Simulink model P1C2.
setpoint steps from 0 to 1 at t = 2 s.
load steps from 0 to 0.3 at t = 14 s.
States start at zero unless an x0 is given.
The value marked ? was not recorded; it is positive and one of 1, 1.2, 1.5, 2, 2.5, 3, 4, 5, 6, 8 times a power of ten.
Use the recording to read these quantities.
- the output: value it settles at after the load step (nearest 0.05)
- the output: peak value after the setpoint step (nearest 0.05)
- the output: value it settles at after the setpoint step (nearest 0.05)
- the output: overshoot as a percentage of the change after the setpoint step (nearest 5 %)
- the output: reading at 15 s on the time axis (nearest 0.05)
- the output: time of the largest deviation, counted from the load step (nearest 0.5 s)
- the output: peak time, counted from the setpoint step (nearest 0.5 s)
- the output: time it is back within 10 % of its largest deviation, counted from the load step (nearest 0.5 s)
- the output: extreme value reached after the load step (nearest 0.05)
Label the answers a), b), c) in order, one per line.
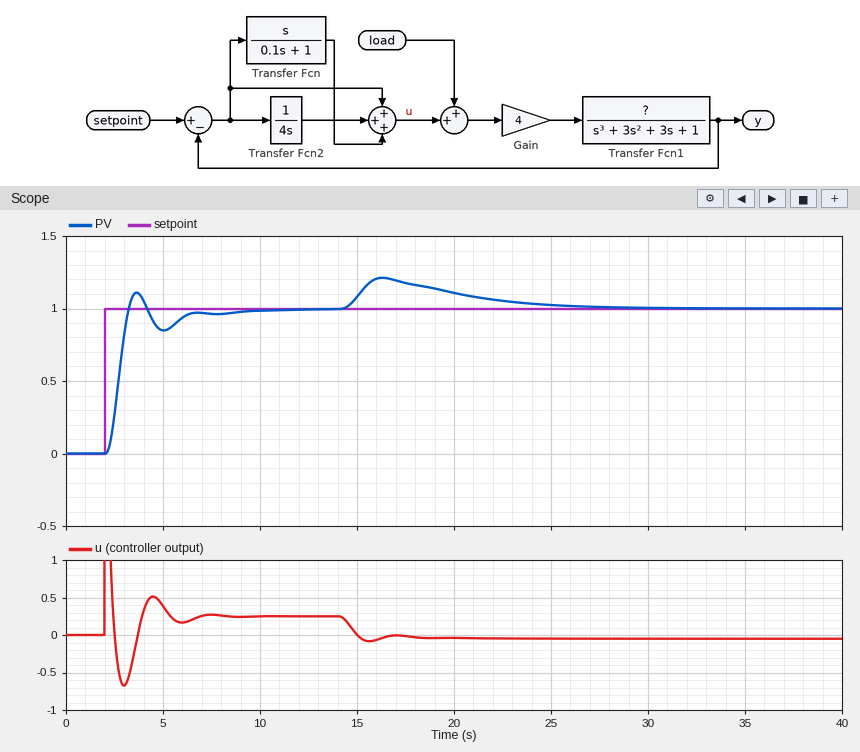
a) 1.00
b) 1.10
c) 1.00
d) 10 %
e) 1.10
f) 2.5 s
g) 1.5 s
h) 11.5 s
i) 1.20
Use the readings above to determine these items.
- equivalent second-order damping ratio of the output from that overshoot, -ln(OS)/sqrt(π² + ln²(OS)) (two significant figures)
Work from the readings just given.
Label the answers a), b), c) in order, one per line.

a) 0.59
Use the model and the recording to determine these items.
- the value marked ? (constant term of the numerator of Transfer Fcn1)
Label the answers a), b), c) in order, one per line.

a) 1
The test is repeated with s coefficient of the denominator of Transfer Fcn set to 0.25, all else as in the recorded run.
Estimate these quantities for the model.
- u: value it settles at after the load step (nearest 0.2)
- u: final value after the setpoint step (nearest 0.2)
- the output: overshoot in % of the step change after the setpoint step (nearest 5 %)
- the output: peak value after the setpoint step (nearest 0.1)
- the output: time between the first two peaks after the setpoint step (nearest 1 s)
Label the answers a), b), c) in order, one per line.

a) 0.0
b) 0.2
c) 25 %
d) 1.2
e) 3 s
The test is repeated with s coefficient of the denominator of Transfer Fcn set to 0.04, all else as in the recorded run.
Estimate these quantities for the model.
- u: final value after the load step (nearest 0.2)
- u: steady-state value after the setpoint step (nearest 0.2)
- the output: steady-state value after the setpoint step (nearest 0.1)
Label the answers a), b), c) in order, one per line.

a) 0.0
b) 0.2
c) 1.0
